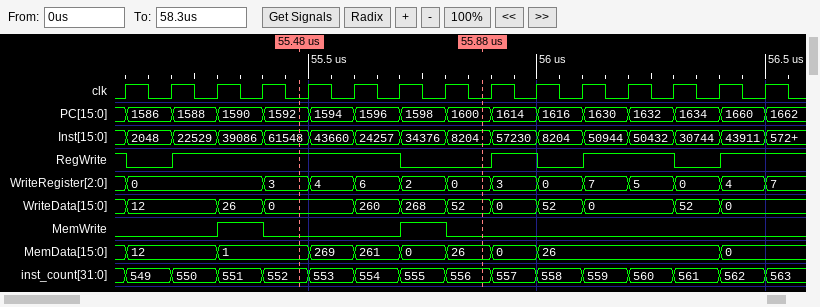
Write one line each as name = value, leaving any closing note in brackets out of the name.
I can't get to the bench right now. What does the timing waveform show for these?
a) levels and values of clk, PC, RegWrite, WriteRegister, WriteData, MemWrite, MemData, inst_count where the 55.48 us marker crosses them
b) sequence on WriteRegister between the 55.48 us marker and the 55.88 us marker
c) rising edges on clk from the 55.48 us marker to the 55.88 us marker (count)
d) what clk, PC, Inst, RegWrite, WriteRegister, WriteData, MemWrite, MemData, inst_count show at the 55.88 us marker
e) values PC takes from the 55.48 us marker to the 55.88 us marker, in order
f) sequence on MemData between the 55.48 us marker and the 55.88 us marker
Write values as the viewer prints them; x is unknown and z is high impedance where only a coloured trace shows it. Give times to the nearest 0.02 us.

levels and values of clk, PC, RegWrite, WriteRegister, WriteData, MemWrite, MemData, inst_count where the 55.48 us marker crosses them = clk=0, PC=1592, RegWrite=1, WriteRegister=3, WriteData=0, MemWrite=0, MemData=1, inst_count=552
sequence on WriteRegister between the 55.48 us marker and the 55.88 us marker = 3, 4, 6, 2, 0
rising edges on clk from the 55.48 us marker to the 55.88 us marker = 4
what clk, PC, Inst, RegWrite, WriteRegister, WriteData, MemWrite, MemData, inst_count show at the 55.88 us marker = clk=0, PC=1600, Inst=8204, RegWrite=0, WriteRegister=0, WriteData=52, MemWrite=0, MemData=26, inst_count=556
values PC takes from the 55.48 us marker to the 55.88 us marker, in order = 1592, 1594, 1596, 1598, 1600
sequence on MemData between the 55.48 us marker and the 55.88 us marker = 1, 269, 261, 0, 26
